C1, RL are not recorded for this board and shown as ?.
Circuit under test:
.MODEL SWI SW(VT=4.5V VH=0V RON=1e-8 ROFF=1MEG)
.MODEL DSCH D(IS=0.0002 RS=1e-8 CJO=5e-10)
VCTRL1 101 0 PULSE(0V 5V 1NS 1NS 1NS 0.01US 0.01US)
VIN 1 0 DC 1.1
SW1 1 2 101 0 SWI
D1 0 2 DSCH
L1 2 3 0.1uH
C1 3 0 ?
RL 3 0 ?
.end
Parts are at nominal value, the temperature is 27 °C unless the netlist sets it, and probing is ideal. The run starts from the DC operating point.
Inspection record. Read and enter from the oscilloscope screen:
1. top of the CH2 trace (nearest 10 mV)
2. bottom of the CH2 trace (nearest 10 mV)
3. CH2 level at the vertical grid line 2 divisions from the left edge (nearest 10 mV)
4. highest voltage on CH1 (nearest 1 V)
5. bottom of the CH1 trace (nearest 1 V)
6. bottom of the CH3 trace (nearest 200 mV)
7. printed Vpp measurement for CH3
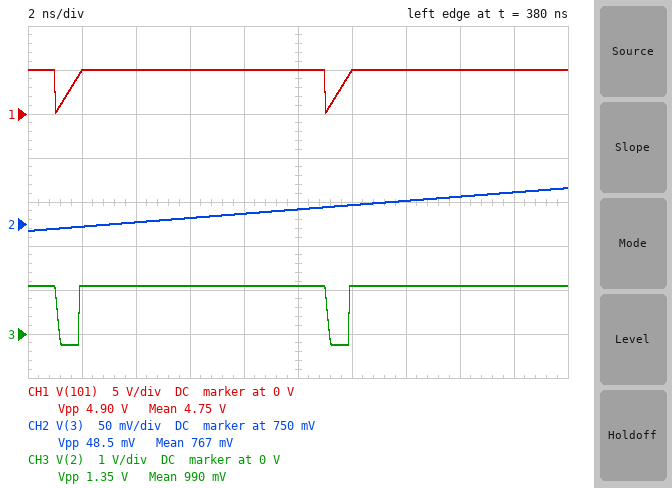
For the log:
790 mV
740 mV
750 mV
5 V
0 V
-200 mV
1.35 V
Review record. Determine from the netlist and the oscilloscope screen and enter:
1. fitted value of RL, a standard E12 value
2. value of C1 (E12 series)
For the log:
0.56 Ω
560 nF
